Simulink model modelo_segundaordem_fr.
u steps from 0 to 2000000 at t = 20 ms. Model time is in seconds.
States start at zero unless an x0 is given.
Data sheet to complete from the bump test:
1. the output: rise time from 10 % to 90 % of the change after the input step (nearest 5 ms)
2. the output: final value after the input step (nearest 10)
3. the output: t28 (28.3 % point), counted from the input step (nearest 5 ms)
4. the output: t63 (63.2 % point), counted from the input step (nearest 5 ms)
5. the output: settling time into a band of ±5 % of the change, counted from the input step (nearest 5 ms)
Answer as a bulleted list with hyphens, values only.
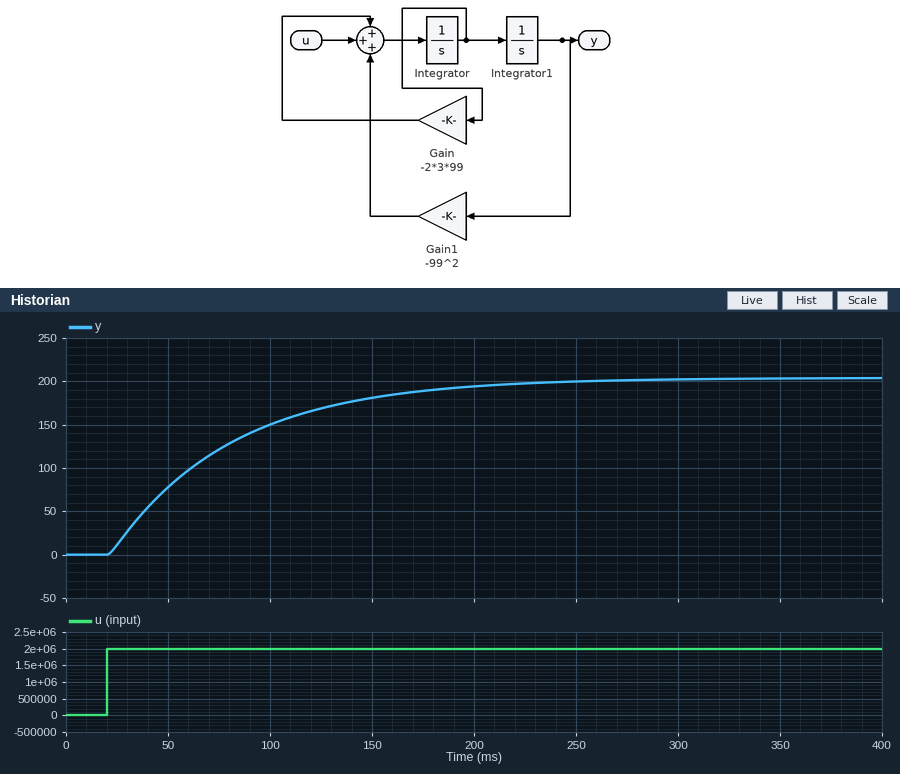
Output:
- 130 ms
- 200
- 20 ms
- 60 ms
- 180 ms
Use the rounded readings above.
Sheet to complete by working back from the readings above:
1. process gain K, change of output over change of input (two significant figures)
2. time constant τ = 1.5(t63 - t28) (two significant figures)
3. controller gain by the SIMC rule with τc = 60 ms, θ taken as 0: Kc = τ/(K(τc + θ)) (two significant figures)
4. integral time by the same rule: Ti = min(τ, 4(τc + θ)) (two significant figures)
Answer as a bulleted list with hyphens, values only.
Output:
- 0.00010
- 60 ms
- 10000
- 60 ms
